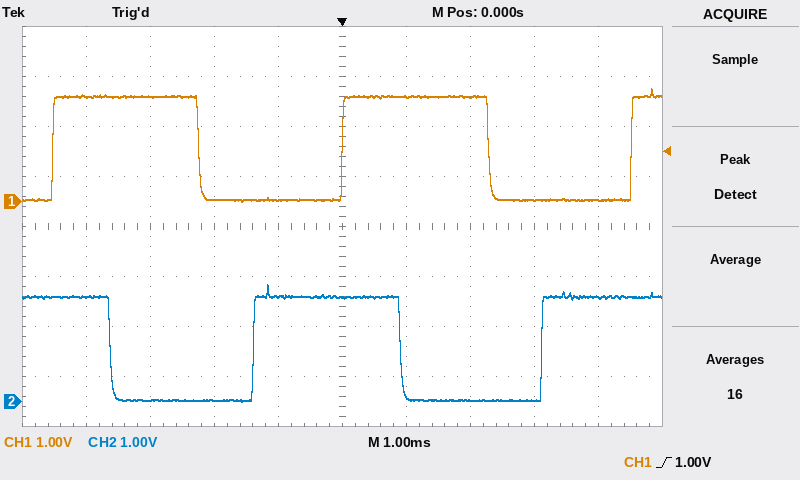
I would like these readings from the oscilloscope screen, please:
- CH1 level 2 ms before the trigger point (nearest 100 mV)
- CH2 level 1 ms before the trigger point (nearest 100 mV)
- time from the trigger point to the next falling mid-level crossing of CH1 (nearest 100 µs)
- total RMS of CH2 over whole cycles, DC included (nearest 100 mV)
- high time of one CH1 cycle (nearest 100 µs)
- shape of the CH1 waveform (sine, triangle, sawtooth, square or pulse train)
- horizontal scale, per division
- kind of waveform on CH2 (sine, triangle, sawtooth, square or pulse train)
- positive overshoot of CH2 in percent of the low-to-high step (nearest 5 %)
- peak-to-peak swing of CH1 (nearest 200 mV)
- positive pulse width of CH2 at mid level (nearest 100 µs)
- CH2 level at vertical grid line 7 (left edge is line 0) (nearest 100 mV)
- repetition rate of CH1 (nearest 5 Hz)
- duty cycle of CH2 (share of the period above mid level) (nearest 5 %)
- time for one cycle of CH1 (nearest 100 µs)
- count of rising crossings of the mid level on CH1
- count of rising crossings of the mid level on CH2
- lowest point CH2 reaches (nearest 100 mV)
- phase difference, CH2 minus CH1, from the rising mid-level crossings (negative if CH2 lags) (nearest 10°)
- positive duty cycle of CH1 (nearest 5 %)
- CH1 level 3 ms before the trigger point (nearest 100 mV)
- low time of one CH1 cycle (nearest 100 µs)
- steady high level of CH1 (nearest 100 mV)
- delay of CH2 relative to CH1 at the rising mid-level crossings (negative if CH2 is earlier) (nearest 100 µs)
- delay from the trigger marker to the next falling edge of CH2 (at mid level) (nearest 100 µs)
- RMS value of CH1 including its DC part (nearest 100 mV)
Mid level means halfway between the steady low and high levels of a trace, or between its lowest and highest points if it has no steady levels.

0.0 V
2.1 V
2.3 ms
1.5 V
2.3 ms
square
1 ms
square
10 %
2.2 V
2.3 ms
0.0 V
220 Hz
50 %
4.5 ms
3
2
0.0 V
+110°
50 %
2.1 V
2.2 ms
2.1 V
-1.4 ms
900 µs
1.5 V
